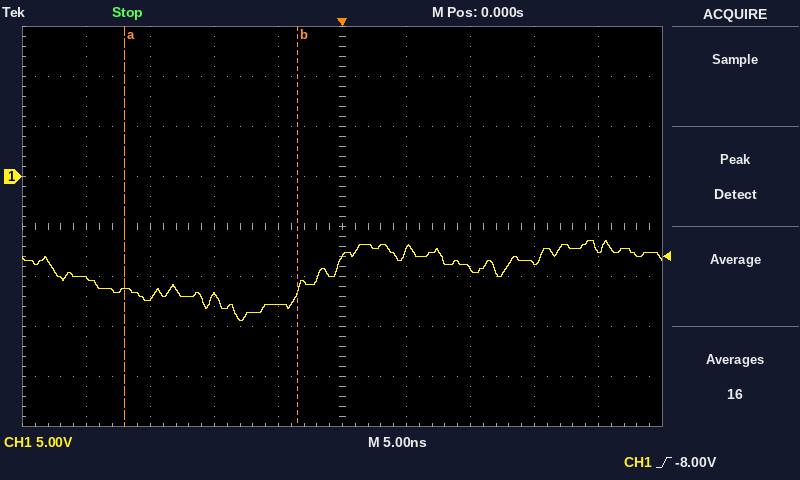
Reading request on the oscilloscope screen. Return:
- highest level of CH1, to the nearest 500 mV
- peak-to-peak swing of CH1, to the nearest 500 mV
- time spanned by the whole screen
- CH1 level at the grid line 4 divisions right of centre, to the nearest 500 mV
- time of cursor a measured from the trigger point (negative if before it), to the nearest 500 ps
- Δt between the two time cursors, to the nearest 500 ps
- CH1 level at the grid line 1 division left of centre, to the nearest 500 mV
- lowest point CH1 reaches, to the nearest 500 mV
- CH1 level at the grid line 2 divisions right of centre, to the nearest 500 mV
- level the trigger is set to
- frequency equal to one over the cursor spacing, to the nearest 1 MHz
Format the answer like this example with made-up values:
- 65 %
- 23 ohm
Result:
- -6.5 V
- 8.0 V
- 50 ns
- -7.5 V
- -17.0 ns
- 13.5 ns
- -13.0 V
- -14.5 V
- -9.0 V
- -8.00 V
- 74 MHz
